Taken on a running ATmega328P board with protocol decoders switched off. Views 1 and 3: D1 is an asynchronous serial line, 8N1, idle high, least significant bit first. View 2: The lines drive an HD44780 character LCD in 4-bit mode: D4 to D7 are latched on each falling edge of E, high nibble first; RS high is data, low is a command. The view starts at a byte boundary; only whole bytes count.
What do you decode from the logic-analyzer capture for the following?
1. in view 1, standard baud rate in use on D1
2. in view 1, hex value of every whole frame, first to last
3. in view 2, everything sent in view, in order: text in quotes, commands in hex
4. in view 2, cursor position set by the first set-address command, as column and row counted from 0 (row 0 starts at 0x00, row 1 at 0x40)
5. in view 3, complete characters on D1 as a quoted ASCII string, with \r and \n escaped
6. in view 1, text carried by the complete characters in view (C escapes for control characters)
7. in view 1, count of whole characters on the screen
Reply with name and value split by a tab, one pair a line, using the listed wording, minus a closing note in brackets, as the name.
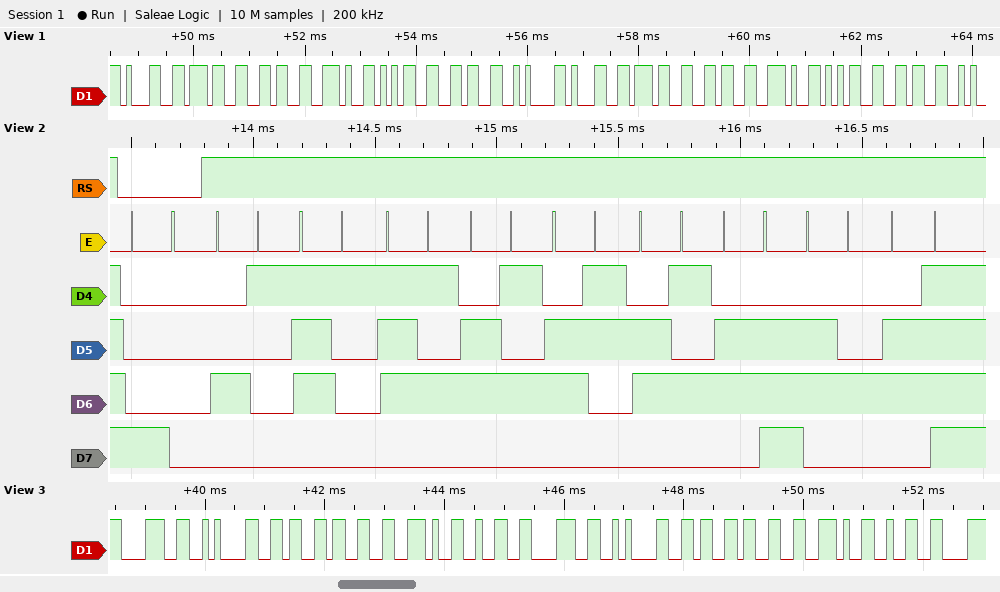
in view 1, standard baud rate in use on D1	9600 baud
in view 1, hex value of every whole frame, first to last	0x31 0x37 0x36 0x2E 0x35 0x36 0x0A 0x31 0x37 0x36 0x2E 0x35 0x36
in view 2, everything sent in view, in order: text in quotes, commands in hex	0x80 "Aquecendo"
in view 2, cursor position set by the first set-address command, as column and row counted from 0	column 0, row 0
in view 3, complete characters on D1 as a quoted ASCII string, with \r and \n escaped	"8\n63.28\n63.2"
in view 1, text carried by the complete characters in view	"176.56\n176.56"
in view 1, count of whole characters on the screen	13
